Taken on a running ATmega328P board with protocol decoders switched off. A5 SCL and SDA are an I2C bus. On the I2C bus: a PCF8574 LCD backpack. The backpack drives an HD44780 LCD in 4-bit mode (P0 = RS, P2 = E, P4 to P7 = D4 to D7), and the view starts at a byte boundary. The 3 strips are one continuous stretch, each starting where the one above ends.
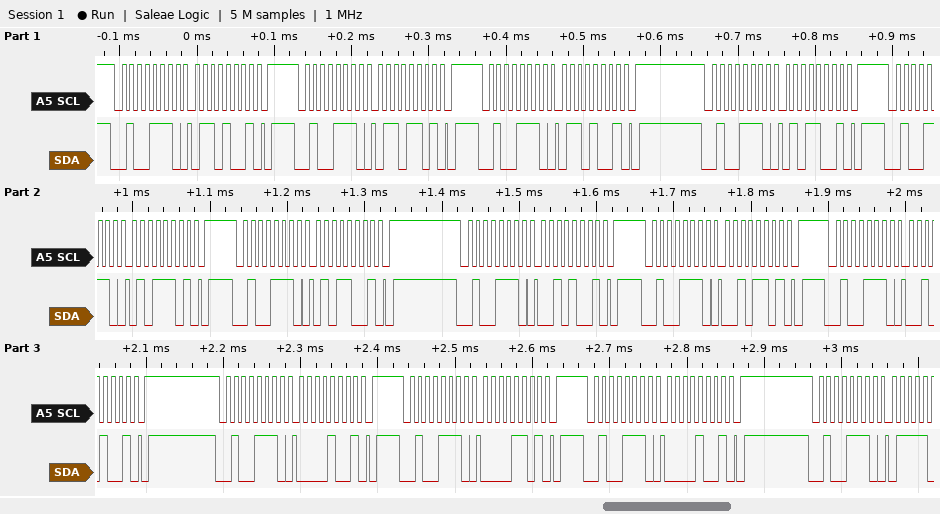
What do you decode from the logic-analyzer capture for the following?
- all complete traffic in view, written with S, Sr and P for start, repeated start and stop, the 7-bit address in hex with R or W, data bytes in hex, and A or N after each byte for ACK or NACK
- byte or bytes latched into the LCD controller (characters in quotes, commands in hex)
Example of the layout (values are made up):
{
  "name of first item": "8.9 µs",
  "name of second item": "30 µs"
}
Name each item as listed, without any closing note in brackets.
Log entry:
{
  "all complete traffic in view, written with S, Sr and P for start, repeated start and stop, the 7-bit address in hex with R or W, data bytes in hex, and A or N after each byte for ACK or NACK": "S 27W A 69 A P S 27W A 6D A P S 27W A 69 A P S 27W A 59 A P S 27W A 5D A P S 27W A 59 A P S 27W A 29 A P S 27W A 2D A P S 27W A 29 A P S 27W A 09 A P S 27W A 0D A P S 27W A 09 A P S 27W A",
  "byte or bytes latched into the LCD controller": "'e' ' '"
}
